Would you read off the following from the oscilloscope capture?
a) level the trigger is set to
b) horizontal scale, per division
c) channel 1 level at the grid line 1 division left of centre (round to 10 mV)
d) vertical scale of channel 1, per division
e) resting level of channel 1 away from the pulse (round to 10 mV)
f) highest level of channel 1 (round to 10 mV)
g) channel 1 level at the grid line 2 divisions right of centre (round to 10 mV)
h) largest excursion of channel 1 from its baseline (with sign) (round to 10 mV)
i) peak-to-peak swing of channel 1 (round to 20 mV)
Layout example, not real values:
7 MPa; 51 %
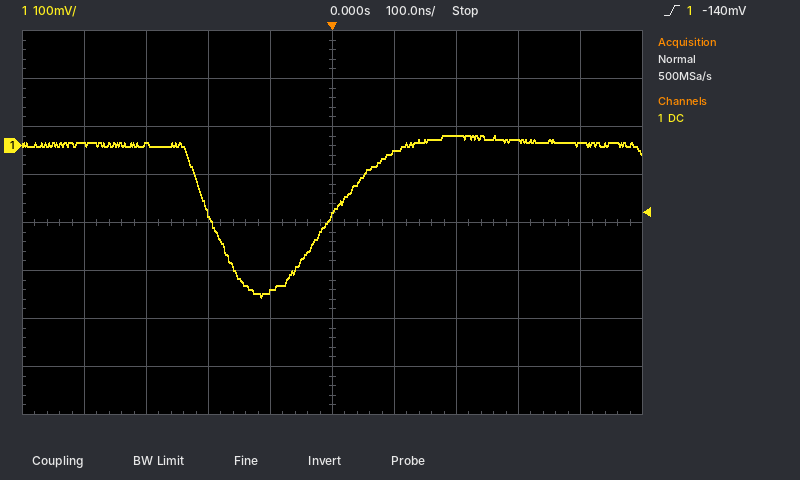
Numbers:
-140 mV; 100 ns; -300 mV; 100 mV; 0 mV; 20 mV; 20 mV; -320 mV; 340 mV
